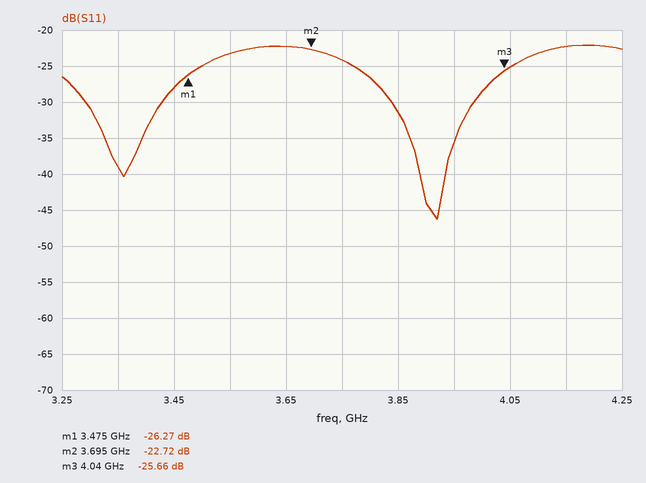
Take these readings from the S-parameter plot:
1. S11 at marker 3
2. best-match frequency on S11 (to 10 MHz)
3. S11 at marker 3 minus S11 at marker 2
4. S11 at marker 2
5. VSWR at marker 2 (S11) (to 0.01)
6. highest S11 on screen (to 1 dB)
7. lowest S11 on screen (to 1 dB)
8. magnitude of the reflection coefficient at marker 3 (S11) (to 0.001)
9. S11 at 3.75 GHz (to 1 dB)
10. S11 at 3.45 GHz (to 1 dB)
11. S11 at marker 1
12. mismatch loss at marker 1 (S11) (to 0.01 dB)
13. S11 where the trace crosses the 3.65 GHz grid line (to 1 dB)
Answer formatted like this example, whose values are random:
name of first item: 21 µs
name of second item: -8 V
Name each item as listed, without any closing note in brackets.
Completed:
S11 at marker 3: -25.66 dB
best-match frequency on S11: 3.92 GHz
S11 at marker 3 minus S11 at marker 2: -2.94 dB
S11 at marker 2: -22.72 dB
VSWR at marker 2 (S11): 1.16
highest S11 on screen: -22 dB
lowest S11 on screen: -46 dB
magnitude of the reflection coefficient at marker 3 (S11): 0.052
S11 at 3.75 GHz: -24 dB
S11 at 3.45 GHz: -28 dB
S11 at marker 1: -26.27 dB
mismatch loss at marker 1 (S11): 0.01 dB
S11 where the trace crosses the 3.65 GHz grid line: -22 dB
